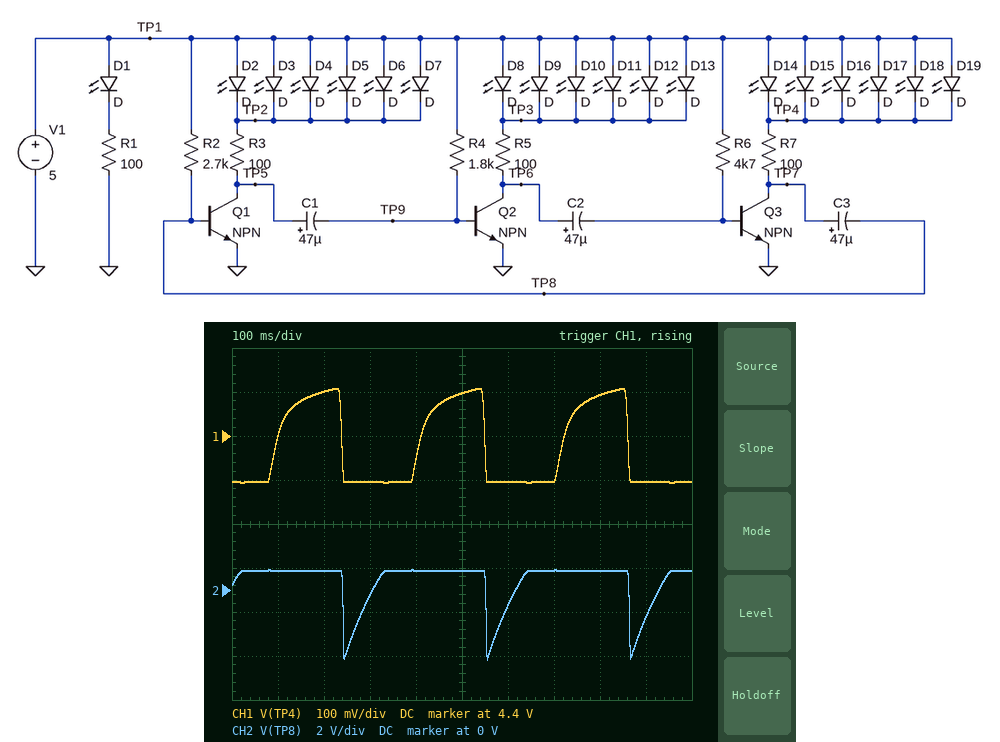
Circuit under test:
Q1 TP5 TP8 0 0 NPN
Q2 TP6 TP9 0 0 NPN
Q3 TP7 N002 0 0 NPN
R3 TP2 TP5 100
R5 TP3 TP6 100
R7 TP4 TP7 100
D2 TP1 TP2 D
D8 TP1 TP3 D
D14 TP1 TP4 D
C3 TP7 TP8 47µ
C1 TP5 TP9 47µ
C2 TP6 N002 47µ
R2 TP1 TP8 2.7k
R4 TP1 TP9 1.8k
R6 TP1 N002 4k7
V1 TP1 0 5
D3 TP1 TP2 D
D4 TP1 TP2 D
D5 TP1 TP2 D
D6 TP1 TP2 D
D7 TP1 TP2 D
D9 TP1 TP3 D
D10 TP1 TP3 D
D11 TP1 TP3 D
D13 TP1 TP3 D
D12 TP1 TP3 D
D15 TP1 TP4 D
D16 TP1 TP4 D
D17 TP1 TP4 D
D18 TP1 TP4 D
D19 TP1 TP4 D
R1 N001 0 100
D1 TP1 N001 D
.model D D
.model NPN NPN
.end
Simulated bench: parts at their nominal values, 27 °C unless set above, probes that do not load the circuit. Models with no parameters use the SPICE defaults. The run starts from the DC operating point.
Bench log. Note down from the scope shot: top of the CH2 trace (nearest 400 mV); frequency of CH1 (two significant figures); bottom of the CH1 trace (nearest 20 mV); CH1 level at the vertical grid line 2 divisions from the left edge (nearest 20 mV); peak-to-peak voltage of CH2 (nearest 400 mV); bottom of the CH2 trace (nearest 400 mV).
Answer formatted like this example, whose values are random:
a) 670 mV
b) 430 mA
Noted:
a) 800 mV
b) 3.2 Hz
c) 4.30 V
d) 4.50 V
e) 4.0 V
f) -3.2 V
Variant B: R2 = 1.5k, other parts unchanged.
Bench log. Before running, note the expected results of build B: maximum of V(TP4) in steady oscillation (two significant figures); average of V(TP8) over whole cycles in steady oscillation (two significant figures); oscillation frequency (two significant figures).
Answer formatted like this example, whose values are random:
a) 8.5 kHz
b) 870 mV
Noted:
a) 4.5 V
b) 560 mV
c) 3.7 Hz
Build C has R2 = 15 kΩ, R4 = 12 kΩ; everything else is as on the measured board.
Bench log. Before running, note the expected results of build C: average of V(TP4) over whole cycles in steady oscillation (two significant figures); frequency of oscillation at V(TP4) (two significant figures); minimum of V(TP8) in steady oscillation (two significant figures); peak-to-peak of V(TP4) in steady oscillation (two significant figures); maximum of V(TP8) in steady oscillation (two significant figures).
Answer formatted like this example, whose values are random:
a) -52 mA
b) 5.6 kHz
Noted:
a) 4.3 V
b) 840 mHz
c) -3.4 V
d) 170 mV
e) 880 mV
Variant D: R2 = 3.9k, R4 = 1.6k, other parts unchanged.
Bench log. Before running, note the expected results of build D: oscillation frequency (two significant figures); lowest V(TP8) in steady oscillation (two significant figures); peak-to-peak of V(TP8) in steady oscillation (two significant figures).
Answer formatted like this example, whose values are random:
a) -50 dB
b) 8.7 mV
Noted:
a) 2.9 Hz
b) -3.3 V
c) 4.2 V
